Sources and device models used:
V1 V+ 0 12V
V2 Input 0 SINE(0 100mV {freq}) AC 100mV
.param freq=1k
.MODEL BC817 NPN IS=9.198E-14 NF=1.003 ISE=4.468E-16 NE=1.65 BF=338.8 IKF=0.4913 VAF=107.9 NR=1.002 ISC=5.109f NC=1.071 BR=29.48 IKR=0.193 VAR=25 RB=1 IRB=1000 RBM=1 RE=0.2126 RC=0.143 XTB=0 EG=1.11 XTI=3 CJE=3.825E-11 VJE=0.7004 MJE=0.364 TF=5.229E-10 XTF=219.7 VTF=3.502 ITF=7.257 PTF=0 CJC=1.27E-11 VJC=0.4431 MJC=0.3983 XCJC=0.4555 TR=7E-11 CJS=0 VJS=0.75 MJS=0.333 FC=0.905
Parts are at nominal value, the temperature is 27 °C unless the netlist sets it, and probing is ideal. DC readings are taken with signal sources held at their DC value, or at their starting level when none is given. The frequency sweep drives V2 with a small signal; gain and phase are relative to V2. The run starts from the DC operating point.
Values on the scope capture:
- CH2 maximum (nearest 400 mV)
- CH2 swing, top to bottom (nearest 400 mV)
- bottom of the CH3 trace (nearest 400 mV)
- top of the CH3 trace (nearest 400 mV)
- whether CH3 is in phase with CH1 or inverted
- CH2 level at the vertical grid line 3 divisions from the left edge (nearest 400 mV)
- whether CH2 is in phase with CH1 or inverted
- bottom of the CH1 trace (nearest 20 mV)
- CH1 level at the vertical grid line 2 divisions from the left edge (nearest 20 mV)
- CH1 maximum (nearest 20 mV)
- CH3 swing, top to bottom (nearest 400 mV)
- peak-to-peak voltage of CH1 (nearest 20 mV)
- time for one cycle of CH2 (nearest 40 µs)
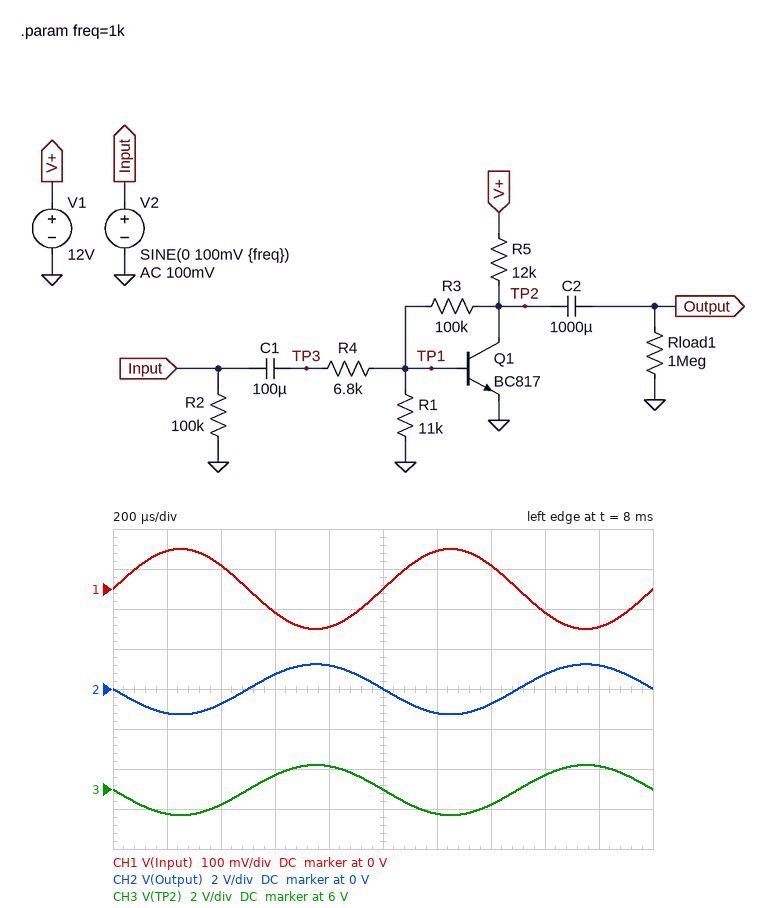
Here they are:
1.2 V
2.4 V
4.8 V
7.2 V
inverted
800 mV
inverted
-100 mV
60 mV
100 mV
2.4 V
200 mV
1.00 ms
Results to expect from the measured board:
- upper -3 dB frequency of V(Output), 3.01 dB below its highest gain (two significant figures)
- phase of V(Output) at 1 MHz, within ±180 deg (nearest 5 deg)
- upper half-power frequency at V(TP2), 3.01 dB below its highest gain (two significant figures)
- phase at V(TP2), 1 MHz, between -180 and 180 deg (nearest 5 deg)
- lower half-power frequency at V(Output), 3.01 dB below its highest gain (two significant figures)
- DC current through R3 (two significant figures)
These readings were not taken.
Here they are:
370 kHz
110 deg
370 kHz
110 deg
220 mHz
54 µA
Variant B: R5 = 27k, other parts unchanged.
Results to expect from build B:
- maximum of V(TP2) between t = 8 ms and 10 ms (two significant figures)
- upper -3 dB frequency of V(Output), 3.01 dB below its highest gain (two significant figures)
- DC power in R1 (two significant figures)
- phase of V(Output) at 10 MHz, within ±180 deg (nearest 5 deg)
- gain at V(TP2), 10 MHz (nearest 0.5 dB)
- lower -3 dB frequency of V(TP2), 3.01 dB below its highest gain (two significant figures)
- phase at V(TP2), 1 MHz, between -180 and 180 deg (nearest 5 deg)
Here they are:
6.9 V
360 kHz
28 µW
60 deg
-8.0 dB
210 mHz
105 deg
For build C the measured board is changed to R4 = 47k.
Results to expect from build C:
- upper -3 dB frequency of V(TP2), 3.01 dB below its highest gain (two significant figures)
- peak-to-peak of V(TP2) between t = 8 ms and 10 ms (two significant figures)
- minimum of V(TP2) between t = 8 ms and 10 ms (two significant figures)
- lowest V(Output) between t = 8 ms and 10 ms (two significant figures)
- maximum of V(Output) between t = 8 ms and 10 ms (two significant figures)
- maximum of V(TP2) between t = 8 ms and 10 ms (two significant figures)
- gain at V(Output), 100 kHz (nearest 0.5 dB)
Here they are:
350 kHz
390 mV
5.8 V
-190 mV
190 mV
6.2 V
5.5 dB
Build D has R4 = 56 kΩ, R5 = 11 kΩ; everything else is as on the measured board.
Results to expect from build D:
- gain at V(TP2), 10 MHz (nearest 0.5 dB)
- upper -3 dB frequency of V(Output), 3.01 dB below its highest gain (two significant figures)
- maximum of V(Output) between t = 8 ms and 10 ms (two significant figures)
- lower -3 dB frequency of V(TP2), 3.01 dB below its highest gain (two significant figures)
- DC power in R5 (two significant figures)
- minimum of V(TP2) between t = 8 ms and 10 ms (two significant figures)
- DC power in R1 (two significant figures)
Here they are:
-25.0 dB
350 kHz
160 mV
28 mHz
3.3 mW
5.8 V
31 µW
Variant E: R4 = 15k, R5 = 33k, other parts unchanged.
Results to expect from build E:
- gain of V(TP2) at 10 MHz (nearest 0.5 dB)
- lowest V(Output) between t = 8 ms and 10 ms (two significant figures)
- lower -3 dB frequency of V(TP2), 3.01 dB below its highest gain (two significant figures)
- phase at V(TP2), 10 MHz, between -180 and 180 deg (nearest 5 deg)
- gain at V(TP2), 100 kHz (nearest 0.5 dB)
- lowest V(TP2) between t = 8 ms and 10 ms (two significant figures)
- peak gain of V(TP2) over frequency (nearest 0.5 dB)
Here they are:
-15.5 dB
-590 mV
100 mHz
55 deg
15.0 dB
5.0 V
15.5 dB
